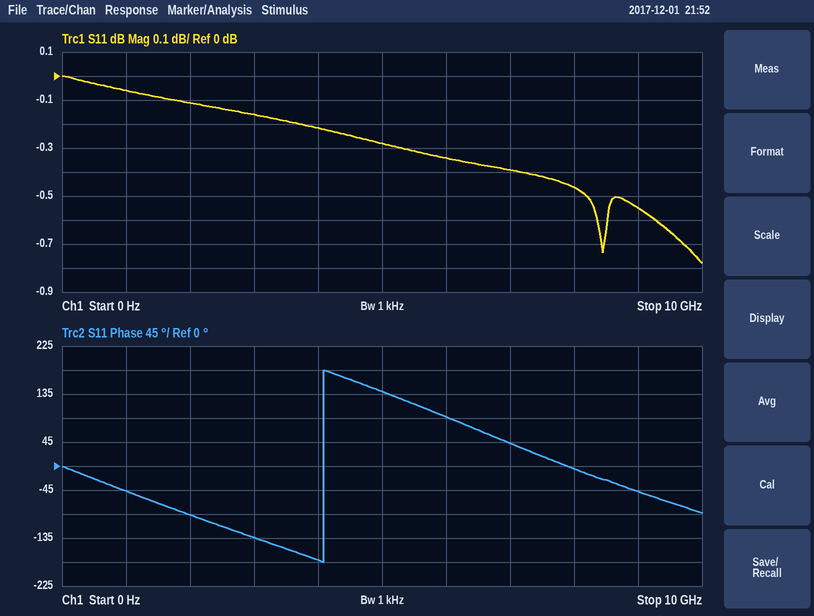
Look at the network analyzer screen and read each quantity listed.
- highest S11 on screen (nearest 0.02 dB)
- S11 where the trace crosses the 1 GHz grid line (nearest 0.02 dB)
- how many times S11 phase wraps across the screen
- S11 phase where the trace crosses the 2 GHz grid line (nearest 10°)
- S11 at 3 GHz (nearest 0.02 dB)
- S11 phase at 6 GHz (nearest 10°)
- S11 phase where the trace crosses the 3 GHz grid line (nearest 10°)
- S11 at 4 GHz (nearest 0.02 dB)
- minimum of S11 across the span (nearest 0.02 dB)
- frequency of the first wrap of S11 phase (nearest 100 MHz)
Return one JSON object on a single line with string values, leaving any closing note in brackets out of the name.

{"highest S11 on screen": "0.00 dB", "S11 where the trace crosses the 1 GHz grid line": "-0.06 dB", "how many times S11 phase wraps across the screen": "1", "S11 phase where the trace crosses the 2 GHz grid line": "-90°", "S11 at 3 GHz": "-0.16 dB", "S11 phase at 6 GHz": "90°", "S11 phase where the trace crosses the 3 GHz grid line": "-130°", "S11 at 4 GHz": "-0.22 dB", "minimum of S11 across the span": "-0.78 dB", "frequency of the first wrap of S11 phase": "4.1 GHz"}
